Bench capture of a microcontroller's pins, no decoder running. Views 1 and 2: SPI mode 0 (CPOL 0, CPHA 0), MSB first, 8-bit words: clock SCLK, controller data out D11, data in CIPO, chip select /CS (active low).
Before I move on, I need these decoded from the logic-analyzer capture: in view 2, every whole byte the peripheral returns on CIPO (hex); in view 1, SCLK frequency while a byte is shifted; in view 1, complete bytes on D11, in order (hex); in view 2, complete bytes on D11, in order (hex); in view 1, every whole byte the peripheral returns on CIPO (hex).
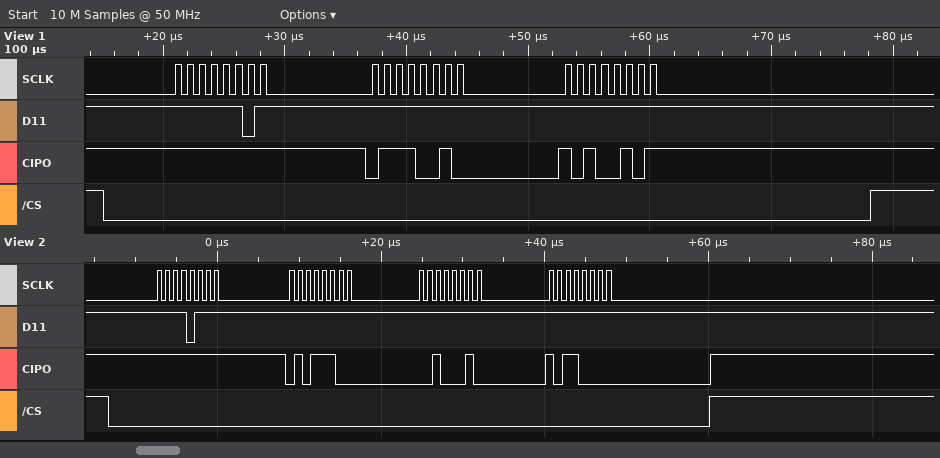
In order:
FF 5C 22 B0
1 MHz
FD FF FF
F7 FF FF FF
FF 72 A5
